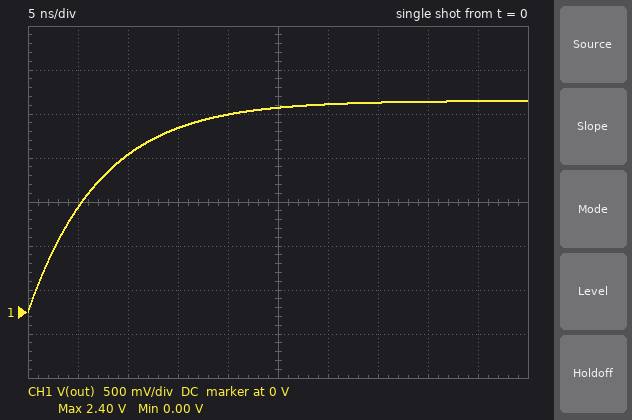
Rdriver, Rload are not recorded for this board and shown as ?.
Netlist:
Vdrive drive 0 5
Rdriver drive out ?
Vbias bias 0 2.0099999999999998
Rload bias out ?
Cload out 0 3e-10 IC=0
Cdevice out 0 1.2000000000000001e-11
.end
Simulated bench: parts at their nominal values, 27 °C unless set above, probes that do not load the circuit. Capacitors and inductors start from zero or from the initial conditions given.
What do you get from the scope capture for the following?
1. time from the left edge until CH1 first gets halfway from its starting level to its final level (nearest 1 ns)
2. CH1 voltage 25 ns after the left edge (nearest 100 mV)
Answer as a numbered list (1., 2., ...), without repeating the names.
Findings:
1. 5 ns
2. 2.3 V
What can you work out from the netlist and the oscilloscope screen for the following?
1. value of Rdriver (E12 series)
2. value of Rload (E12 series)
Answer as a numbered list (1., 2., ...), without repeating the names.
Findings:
1. 180 Ω
2. 27 Ω
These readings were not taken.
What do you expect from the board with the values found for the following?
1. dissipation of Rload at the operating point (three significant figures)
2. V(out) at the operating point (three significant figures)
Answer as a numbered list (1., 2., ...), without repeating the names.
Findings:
1. 5.63 mW
2. 2.40 V
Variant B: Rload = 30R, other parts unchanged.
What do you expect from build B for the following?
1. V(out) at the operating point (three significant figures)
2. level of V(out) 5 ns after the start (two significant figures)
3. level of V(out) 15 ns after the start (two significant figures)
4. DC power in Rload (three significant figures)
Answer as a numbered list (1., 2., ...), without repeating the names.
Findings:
1. 2.44 V
2. 1.1 V
3. 2.1 V
4. 6.08 mW
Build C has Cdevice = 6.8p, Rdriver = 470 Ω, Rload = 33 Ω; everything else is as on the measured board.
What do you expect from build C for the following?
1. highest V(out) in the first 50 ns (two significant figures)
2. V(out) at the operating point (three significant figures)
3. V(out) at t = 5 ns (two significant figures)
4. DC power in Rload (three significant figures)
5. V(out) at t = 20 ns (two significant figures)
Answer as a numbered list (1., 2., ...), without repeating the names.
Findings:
1. 2.2 V
2. 2.21 V
3. 910 mV
4. 1.17 mW
5. 1.9 V
